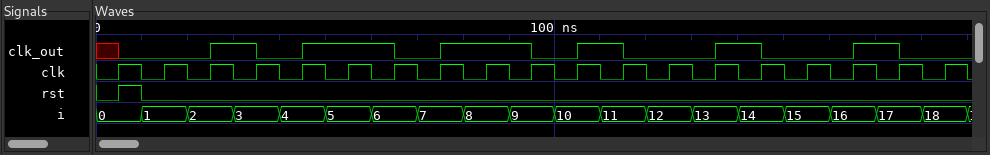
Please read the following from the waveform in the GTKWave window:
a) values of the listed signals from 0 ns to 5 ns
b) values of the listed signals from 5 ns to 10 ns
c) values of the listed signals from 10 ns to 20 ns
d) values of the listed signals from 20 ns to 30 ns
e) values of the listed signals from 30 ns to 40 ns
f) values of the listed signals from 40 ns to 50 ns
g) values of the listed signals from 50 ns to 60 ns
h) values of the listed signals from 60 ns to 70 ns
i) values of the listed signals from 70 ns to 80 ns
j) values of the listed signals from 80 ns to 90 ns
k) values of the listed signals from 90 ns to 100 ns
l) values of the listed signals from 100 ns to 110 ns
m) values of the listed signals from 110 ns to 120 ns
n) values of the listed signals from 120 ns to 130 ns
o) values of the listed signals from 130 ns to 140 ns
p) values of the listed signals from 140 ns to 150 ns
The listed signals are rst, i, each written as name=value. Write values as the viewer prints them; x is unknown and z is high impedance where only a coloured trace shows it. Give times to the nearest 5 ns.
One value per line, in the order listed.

rst=0, i=0
rst=1, i=0
rst=0, i=1
rst=0, i=2
rst=0, i=3
rst=0, i=4
rst=0, i=5
rst=0, i=6
rst=0, i=7
rst=0, i=8
rst=0, i=9
rst=0, i=10
rst=0, i=11
rst=0, i=12
rst=0, i=13
rst=0, i=14
